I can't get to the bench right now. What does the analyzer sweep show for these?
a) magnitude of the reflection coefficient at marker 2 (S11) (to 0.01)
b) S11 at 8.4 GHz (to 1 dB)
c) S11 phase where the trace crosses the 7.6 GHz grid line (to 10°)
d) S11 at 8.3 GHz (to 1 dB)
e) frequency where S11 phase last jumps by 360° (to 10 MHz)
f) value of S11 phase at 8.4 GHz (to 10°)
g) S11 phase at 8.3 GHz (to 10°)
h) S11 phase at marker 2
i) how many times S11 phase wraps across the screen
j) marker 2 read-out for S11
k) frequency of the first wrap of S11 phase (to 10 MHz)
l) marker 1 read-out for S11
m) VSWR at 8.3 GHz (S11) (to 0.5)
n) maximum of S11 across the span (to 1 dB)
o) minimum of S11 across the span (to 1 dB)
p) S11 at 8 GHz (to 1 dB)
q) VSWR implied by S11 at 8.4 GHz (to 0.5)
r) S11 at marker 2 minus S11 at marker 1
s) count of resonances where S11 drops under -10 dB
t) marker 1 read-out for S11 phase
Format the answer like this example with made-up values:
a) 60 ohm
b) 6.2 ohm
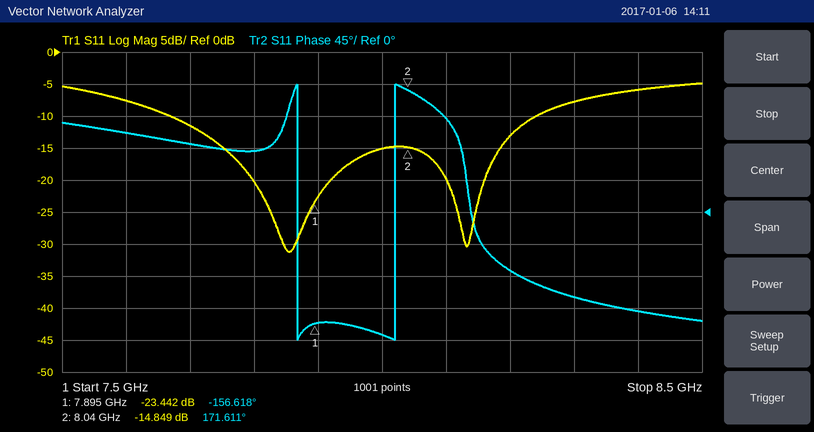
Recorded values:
a) 0.18
b) -6 dB
c) 110°
d) -8 dB
e) 8.02 GHz
f) -140°
g) -120°
h) 171.611°
i) 2
j) -14.849 dB
k) 7.87 GHz
l) -23.442 dB
m) 2.5
n) -5 dB
o) -31 dB
p) -15 dB
q) 3.0
r) 8.593 dB
s) 2
t) -156.618°
